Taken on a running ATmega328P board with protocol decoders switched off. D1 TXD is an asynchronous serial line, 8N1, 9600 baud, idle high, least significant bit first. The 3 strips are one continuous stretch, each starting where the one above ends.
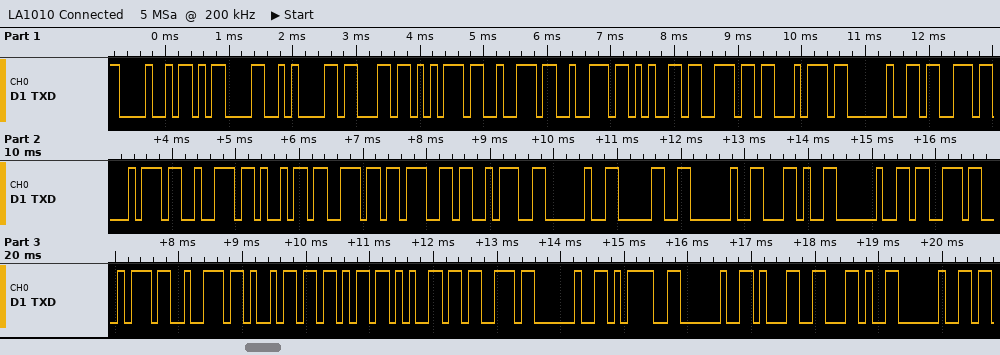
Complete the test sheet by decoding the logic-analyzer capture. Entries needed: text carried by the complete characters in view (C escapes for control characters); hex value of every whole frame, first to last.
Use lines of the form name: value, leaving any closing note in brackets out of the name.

text carried by the complete characters in view: "H\r\ncurrent string: 0 , strikes = 1, "
hex value of every whole frame, first to last: 0x48 0x0D 0x0A 0x63 0x75 0x72 0x72 0x65 0x6E 0x74 0x20 0x73 0x74 0x72 0x69 0x6E 0x67 0x3A 0x20 0x30 0x20 0x2C 0x20 0x73 0x74 0x72 0x69 0x6B 0x65 0x73 0x20 0x3D 0x20 0x31 0x2C 0x20
